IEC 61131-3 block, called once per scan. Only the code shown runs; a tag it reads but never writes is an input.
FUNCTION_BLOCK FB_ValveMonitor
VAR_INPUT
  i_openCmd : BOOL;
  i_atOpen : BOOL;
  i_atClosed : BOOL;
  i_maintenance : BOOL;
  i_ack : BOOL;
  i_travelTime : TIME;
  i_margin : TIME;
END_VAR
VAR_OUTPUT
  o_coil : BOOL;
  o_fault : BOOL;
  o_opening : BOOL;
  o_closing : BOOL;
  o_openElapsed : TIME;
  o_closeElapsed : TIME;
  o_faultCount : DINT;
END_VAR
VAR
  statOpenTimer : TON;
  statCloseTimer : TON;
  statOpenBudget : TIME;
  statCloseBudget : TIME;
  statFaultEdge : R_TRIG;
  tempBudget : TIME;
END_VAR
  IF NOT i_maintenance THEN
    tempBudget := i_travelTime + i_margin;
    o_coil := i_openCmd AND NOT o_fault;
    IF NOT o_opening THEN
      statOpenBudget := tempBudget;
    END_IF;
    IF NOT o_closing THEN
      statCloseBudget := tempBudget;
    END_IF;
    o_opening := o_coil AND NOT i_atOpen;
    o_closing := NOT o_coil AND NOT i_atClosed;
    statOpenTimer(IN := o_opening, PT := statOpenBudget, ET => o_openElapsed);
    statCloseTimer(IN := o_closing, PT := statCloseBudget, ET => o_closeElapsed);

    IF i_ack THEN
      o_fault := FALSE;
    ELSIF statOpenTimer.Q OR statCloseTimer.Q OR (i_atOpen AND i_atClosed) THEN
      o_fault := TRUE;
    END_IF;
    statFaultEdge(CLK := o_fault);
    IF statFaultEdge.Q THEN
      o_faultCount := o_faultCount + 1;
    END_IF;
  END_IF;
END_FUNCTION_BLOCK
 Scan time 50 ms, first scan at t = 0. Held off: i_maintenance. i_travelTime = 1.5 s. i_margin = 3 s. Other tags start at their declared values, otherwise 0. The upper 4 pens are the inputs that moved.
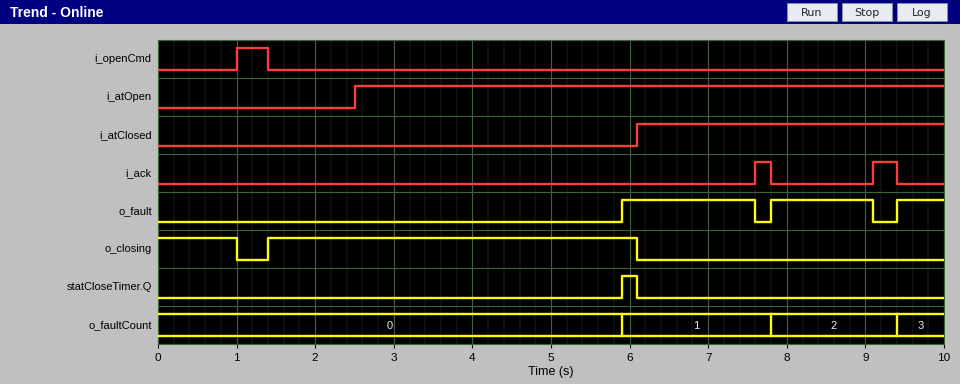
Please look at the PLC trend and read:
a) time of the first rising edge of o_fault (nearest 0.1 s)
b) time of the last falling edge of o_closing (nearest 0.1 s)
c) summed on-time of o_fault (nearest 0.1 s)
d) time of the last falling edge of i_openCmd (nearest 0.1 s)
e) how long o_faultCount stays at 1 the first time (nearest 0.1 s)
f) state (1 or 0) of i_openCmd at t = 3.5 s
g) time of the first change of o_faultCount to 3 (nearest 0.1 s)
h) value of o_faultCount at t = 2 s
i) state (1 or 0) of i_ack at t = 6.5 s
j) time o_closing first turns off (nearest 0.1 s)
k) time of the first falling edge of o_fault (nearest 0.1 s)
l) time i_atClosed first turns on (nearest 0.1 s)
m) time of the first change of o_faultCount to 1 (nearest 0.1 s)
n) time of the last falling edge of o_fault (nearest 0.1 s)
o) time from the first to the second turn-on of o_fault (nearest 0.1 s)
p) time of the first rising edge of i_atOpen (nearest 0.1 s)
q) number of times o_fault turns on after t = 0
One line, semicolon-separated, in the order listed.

5.9 s; 6.1 s; 3.6 s; 1.4 s; 1.9 s; 0; 9.4 s; 0; 0; 1.0 s; 7.6 s; 6.1 s; 5.9 s; 9.1 s; 1.9 s; 2.5 s; 3
